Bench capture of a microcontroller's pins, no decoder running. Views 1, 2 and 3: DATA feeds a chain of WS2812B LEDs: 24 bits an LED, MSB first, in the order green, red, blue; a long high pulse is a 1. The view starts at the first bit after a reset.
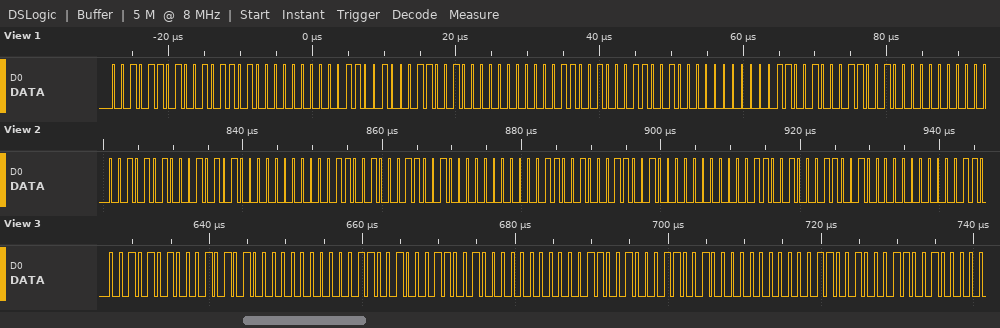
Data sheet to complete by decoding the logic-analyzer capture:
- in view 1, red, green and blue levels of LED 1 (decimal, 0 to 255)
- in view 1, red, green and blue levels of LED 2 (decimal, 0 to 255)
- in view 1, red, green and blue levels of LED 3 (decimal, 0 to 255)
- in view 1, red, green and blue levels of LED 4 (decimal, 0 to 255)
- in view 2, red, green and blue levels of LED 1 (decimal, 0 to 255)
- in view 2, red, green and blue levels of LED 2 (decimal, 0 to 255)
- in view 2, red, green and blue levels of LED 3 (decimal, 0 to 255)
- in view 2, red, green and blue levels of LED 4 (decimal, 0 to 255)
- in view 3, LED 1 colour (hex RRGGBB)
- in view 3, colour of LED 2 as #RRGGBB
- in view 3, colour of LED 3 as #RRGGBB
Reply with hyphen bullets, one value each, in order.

- 45, 45, 0
- 50, 50, 0
- 50, 50, 0
- 50, 50, 0
- 42, 42, 0
- 50, 50, 0
- 50, 50, 0
- 50, 50, 0
- #2A2A00
- #323200
- #323200
